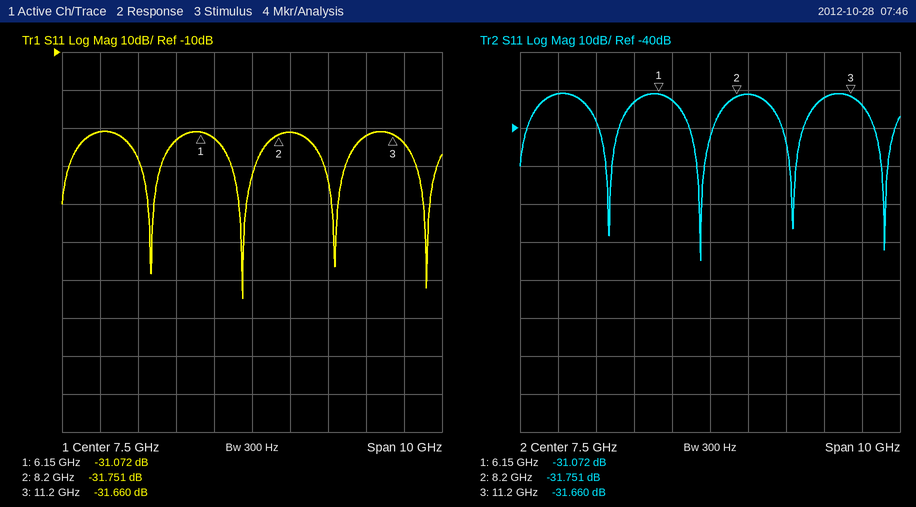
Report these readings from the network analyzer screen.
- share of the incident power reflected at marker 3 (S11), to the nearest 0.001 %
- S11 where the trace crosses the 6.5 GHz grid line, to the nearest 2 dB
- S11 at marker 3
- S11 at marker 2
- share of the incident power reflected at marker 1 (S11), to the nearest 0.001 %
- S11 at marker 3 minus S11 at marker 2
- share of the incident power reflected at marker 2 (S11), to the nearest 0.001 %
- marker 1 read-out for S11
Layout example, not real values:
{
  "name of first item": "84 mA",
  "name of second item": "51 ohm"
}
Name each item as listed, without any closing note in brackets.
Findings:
{
  "share of the incident power reflected at marker 3 (S11), to the nearest 0.001 %": "0.068 %",
  "S11 where the trace crosses the 6.5 GHz grid line, to the nearest 2 dB": "-32 dB",
  "S11 at marker 3": "-31.660 dB",
  "S11 at marker 2": "-31.751 dB",
  "share of the incident power reflected at marker 1 (S11), to the nearest 0.001 %": "0.078 %",
  "S11 at marker 3 minus S11 at marker 2": "0.091 dB",
  "share of the incident power reflected at marker 2 (S11), to the nearest 0.001 %": "0.067 %",
  "marker 1 read-out for S11": "-31.072 dB"
}
